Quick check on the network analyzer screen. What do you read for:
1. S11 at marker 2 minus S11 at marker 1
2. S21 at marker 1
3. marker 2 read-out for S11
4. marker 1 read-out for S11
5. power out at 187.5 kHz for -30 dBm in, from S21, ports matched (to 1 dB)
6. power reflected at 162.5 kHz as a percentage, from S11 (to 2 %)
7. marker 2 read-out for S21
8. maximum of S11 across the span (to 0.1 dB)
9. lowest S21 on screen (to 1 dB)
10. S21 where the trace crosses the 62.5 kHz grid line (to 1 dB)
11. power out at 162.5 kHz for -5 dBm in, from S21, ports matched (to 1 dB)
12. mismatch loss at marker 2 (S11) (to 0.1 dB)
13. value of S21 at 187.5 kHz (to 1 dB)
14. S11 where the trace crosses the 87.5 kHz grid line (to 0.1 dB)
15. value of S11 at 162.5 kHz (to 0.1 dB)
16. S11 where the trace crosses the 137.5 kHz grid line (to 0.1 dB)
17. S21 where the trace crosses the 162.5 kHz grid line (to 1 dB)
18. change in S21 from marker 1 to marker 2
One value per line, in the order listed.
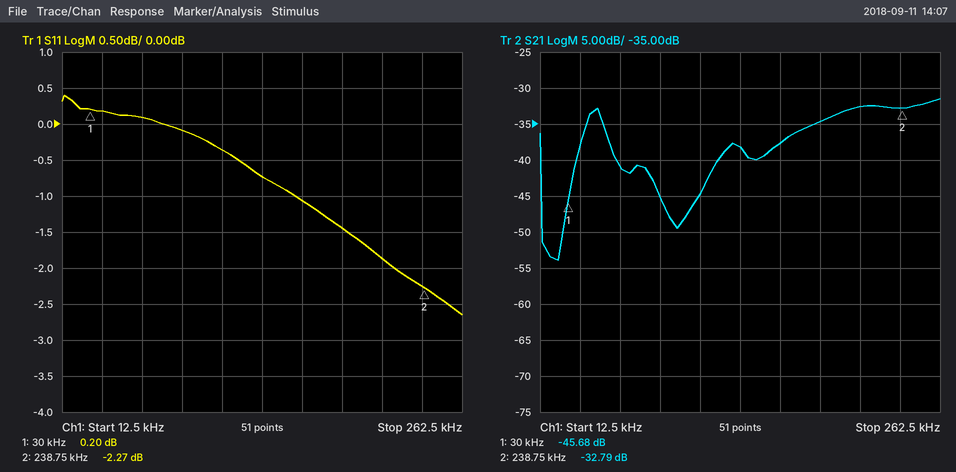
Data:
-2.47 dB
-45.68 dB
-2.27 dB
0.20 dB
-65 dBm
78 %
-32.79 dB
0.4 dB
-54 dB
-41 dB
-43 dBm
3.9 dB
-35 dB
-0.1 dB
-1.1 dB
-0.7 dB
-38 dB
12.89 dB
